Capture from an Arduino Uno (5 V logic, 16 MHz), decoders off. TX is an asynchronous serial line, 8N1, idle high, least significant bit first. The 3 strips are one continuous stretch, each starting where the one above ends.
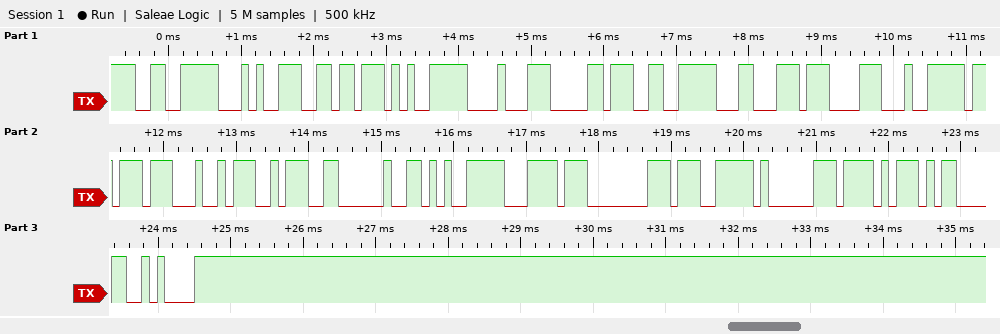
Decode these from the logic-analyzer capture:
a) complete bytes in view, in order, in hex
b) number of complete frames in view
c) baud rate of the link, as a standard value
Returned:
0xE6 0x94 0xB6 0xE5 0x88 0xB0 0xE6 0x8C 0x87 0xE4 0xBB 0xA4 0x3A 0x20 0xE5 0xBC 0x80 0xE7 0x81 0xAF 0x0D 0x0A
22
9600 baud
